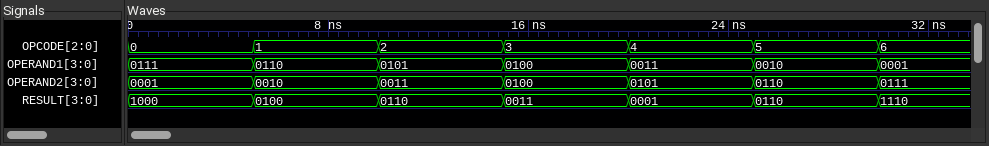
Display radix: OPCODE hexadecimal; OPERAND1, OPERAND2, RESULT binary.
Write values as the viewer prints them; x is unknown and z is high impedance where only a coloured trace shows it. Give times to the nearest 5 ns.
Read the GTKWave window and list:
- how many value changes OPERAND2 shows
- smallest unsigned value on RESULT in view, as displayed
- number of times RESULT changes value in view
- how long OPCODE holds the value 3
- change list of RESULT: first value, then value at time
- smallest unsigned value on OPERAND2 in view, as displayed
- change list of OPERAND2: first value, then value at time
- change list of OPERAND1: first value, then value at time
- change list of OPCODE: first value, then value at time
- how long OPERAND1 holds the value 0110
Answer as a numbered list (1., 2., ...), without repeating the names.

1. 6
2. 0001
3. 6
4. 5 ns
5. 1000, 0100 at 5 ns, 0110 at 10 ns, 0011 at 15 ns, 0001 at 20 ns, 0110 at 25 ns, 1110 at 30 ns
6. 0001
7. 0001, 0010 at 5 ns, 0011 at 10 ns, 0100 at 15 ns, 0101 at 20 ns, 0110 at 25 ns, 0111 at 30 ns
8. 0111, 0110 at 5 ns, 0101 at 10 ns, 0100 at 15 ns, 0011 at 20 ns, 0010 at 25 ns, 0001 at 30 ns
9. 0, 1 at 5 ns, 2 at 10 ns, 3 at 15 ns, 4 at 20 ns, 5 at 25 ns, 6 at 30 ns
10. 5 ns
